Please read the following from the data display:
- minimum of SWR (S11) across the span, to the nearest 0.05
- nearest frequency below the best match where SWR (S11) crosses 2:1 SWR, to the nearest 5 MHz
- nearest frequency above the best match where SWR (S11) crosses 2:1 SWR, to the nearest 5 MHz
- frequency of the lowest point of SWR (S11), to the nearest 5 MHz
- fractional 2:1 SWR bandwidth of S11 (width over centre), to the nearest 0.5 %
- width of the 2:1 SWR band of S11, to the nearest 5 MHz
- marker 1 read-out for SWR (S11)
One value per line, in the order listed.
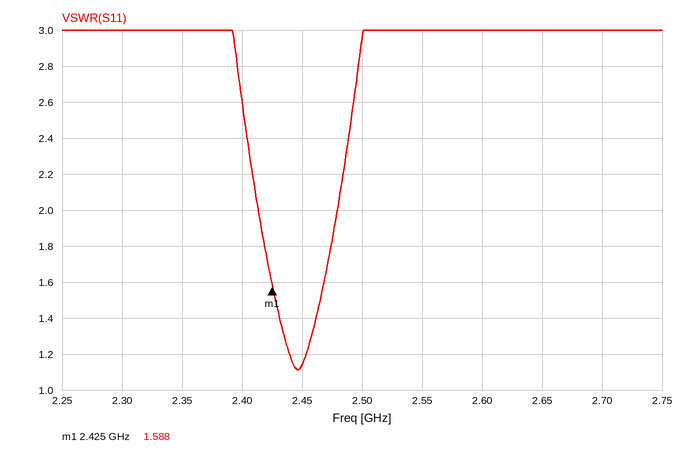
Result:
1.10
2.415 GHz
2.480 GHz
2.445 GHz
2.5 %
65 MHz
1.588
